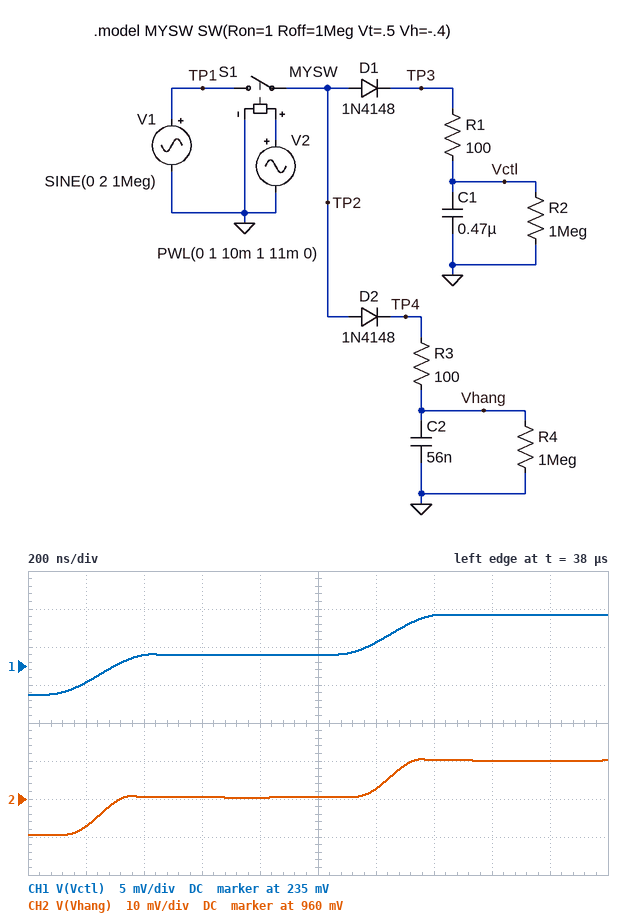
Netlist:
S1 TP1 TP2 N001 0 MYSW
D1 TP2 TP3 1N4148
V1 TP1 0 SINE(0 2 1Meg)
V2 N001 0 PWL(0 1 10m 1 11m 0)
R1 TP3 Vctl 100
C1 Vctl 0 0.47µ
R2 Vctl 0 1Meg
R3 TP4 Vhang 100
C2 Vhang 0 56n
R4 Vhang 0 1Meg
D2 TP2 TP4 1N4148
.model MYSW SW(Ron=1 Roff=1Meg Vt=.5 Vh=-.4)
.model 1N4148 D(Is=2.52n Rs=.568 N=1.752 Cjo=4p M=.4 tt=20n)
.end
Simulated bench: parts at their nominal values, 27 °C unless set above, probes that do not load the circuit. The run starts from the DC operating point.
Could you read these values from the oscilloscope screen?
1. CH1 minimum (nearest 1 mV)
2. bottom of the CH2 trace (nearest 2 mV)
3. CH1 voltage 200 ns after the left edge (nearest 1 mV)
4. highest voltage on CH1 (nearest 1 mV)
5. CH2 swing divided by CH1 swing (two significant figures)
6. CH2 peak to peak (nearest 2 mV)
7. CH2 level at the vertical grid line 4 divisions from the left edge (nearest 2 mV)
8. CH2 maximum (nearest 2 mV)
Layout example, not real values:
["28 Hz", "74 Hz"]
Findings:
["231 mV", "950 mV", "233 mV", "242 mV", "1.9", "20 mV", "960 mV", "970 mV"]
